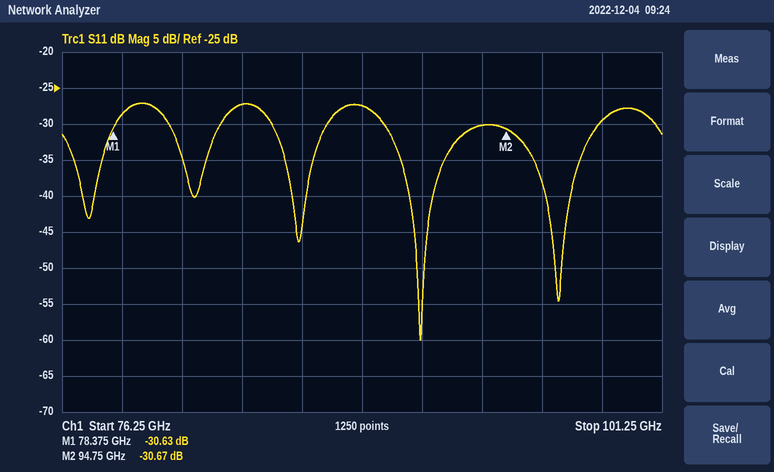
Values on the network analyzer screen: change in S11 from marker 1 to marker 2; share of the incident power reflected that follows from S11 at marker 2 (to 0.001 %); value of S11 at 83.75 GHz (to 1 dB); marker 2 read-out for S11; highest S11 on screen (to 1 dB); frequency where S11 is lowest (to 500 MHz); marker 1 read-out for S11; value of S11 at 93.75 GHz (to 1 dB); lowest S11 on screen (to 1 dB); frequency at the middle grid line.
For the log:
-0.04 dB
0.086 %
-27 dB
-30.67 dB
-27 dB
91.0 GHz
-30.63 dB
-30 dB
-60 dB
88.75 GHz
